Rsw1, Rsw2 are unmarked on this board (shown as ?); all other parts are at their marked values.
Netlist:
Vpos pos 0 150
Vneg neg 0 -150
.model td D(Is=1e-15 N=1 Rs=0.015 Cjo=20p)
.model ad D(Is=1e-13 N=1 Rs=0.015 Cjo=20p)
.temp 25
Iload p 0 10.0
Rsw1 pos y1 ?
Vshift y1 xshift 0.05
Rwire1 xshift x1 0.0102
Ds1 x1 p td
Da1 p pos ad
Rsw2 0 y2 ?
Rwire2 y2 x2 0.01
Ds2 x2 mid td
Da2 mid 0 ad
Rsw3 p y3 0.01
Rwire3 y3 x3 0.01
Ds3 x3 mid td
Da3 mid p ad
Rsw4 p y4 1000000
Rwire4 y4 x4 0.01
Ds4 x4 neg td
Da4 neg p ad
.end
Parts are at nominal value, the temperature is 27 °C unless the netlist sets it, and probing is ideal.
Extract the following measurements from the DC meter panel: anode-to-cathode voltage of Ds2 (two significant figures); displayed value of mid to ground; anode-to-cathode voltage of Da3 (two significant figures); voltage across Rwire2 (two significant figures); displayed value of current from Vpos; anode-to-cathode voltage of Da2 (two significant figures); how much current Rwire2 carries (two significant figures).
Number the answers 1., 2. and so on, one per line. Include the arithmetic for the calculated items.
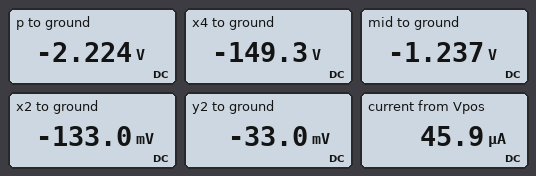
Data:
1. -133 mV - (-1.237 V) = 1.1 V
2. -1.237 V
3. -1.237 V - (-2.224 V) = 990 mV
4. -33 mV - (-133 mV) = 100 mV
5. 45.9 µA
6. -1.237 V = -1.2 V
7. (-33 mV - (-133 mV)) / 10 mΩ = 10 A
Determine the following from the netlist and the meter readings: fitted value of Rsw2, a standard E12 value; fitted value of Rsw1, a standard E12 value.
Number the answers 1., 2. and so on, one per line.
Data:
1. 3.3 mΩ
2. 3.3 MΩ
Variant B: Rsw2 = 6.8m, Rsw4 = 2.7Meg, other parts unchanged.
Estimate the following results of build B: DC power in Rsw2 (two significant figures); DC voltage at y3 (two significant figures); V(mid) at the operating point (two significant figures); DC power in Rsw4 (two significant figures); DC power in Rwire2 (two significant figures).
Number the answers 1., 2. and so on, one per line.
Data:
1. 680 mW
2. -2.3 V
3. -1.3 V
4. 8.0 mW
5. 1.0 W
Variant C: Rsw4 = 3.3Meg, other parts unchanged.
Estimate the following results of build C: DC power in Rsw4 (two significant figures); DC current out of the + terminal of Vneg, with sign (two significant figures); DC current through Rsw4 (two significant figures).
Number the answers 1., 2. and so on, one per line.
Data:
1. 6.6 mW
2. -45 µA
3. 45 µA
